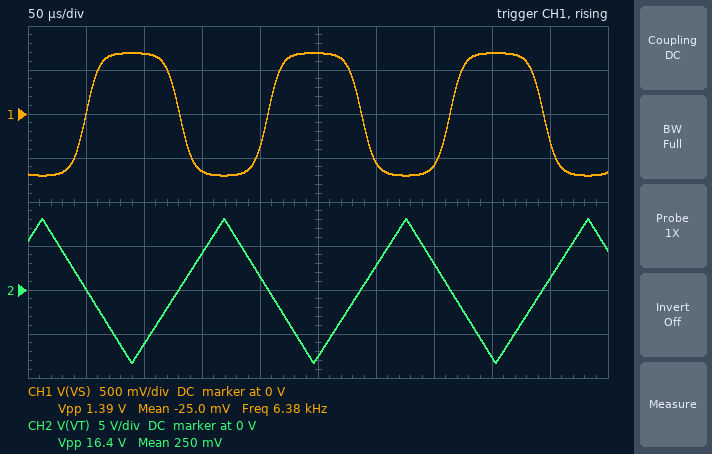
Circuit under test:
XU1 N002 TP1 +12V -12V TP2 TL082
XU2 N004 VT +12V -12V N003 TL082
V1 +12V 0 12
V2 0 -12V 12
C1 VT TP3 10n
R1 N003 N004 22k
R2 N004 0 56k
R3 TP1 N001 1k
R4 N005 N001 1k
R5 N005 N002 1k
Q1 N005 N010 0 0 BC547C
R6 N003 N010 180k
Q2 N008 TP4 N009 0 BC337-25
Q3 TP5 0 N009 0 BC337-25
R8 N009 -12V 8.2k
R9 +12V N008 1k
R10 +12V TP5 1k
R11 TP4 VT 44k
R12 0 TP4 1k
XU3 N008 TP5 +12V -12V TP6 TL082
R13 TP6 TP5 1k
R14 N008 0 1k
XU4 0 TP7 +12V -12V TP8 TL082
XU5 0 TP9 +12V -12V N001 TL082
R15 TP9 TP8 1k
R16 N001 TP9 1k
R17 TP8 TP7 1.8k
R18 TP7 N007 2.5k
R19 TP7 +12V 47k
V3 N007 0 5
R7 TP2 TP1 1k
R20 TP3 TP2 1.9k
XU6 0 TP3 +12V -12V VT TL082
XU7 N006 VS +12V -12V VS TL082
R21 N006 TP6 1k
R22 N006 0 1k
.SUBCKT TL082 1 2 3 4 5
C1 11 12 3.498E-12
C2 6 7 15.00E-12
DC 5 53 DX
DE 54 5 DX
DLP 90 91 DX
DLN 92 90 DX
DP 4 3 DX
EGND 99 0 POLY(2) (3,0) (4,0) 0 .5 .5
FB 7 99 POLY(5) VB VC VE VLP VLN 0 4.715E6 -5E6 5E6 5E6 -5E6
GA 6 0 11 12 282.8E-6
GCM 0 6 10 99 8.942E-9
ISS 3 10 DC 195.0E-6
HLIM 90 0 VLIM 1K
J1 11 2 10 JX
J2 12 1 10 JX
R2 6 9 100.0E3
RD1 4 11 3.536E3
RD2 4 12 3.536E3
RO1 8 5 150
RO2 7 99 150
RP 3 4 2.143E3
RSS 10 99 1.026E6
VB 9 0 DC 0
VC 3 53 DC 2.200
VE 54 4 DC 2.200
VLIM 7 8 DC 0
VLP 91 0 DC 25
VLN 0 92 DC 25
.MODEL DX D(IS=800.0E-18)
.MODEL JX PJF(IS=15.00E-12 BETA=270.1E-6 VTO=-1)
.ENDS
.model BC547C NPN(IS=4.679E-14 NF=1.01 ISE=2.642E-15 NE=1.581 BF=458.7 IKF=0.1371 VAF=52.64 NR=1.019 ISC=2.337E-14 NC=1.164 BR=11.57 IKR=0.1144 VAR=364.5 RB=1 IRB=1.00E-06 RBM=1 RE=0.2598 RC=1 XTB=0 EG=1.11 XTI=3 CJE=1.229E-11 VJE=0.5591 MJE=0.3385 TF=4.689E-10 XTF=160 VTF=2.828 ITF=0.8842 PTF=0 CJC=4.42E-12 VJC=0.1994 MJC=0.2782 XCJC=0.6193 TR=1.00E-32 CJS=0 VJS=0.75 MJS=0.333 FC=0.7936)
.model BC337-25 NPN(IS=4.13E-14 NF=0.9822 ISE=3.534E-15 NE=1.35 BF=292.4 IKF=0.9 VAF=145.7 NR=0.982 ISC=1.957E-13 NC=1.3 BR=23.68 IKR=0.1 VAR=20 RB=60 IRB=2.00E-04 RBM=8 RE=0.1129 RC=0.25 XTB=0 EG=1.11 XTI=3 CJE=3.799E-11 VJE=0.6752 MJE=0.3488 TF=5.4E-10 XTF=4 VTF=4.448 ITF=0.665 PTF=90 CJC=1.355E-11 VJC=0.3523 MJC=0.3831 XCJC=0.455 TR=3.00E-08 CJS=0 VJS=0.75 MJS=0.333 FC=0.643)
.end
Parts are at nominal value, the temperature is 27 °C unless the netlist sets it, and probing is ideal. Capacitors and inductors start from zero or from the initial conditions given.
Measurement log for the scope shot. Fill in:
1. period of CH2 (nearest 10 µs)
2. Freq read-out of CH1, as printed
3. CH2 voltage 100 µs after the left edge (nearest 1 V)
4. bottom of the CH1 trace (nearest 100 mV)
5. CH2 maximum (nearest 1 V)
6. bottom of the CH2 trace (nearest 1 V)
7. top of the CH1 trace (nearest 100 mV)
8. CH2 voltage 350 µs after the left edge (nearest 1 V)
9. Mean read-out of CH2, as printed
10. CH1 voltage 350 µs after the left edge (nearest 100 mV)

160 µs
6.38 kHz
-6 V
-700 mV
8 V
-8 V
700 mV
3 V
250 mV
-600 mV
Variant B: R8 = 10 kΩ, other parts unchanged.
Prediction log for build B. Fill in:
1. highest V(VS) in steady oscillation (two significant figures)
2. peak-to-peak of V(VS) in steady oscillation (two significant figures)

570 mV
1.1 V
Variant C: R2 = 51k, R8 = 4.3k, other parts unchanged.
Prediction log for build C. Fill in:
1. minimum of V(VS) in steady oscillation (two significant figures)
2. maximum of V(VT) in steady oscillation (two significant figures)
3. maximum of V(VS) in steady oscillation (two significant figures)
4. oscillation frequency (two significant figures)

-1.3 V
7.9 V
1.3 V
6.5 kHz
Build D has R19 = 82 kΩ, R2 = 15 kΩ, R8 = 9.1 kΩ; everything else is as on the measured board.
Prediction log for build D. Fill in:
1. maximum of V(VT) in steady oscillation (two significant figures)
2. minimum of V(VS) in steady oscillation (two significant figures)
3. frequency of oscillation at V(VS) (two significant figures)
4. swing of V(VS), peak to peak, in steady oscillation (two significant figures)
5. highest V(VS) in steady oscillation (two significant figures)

4.8 V
-610 mV
10 kHz
1.2 V
610 mV
